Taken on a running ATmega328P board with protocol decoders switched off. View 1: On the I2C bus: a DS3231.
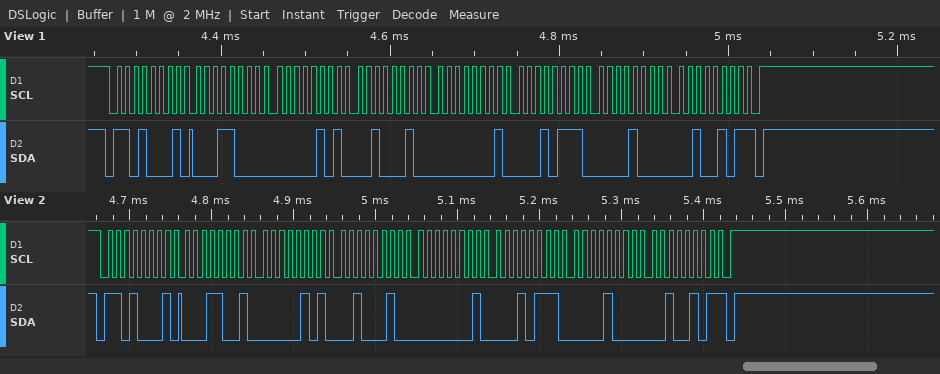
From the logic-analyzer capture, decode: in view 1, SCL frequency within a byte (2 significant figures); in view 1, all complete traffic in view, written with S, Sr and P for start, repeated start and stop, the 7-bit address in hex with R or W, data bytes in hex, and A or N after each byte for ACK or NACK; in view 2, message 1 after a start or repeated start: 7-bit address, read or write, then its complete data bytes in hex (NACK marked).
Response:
100 kHz
S 68R A 18 A 05 A 22 A 01 A 17 A 08 A 25 N P
0x68 read: 19 05 22 01 17 08 25 NACK
